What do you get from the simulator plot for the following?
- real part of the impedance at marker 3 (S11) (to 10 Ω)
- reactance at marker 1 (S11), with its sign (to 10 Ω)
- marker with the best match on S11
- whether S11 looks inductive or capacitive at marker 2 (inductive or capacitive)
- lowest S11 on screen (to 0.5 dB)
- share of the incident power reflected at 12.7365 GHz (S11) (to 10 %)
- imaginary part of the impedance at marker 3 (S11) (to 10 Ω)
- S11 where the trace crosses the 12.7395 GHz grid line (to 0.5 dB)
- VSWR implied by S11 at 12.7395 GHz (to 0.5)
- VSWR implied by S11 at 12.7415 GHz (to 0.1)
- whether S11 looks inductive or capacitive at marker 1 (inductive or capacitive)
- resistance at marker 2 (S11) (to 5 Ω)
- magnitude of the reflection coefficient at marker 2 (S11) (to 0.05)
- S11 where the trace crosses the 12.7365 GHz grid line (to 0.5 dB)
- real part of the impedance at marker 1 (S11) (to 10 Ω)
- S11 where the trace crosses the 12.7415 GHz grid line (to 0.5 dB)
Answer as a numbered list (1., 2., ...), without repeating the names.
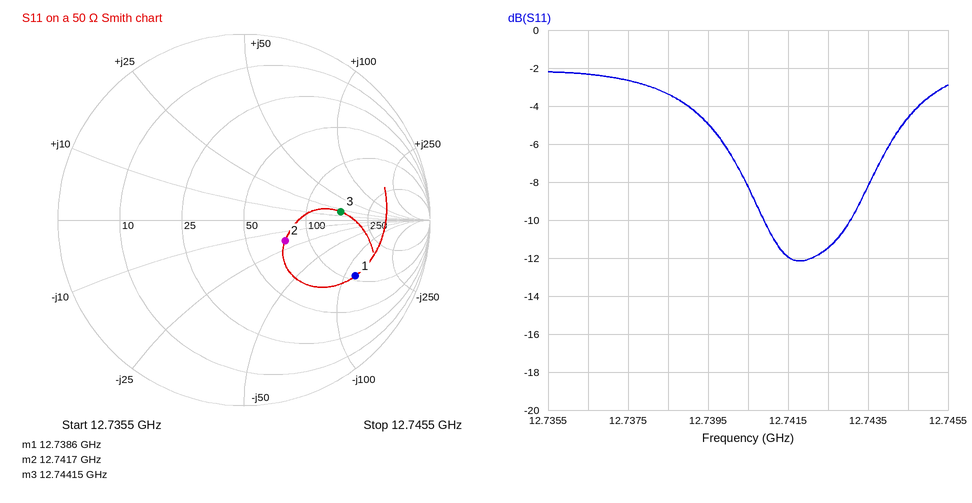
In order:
1. 160 Ω
2. -120 Ω
3. marker 2
4. capacitive
5. -12.0 dB
6. 60 %
7. +20 Ω
8. -5.0 dB
9. 3.5
10. 1.7
11. capacitive
12. 75 Ω
13. 0.25
14. -2.5 dB
15. 110 Ω
16. -12.0 dB
